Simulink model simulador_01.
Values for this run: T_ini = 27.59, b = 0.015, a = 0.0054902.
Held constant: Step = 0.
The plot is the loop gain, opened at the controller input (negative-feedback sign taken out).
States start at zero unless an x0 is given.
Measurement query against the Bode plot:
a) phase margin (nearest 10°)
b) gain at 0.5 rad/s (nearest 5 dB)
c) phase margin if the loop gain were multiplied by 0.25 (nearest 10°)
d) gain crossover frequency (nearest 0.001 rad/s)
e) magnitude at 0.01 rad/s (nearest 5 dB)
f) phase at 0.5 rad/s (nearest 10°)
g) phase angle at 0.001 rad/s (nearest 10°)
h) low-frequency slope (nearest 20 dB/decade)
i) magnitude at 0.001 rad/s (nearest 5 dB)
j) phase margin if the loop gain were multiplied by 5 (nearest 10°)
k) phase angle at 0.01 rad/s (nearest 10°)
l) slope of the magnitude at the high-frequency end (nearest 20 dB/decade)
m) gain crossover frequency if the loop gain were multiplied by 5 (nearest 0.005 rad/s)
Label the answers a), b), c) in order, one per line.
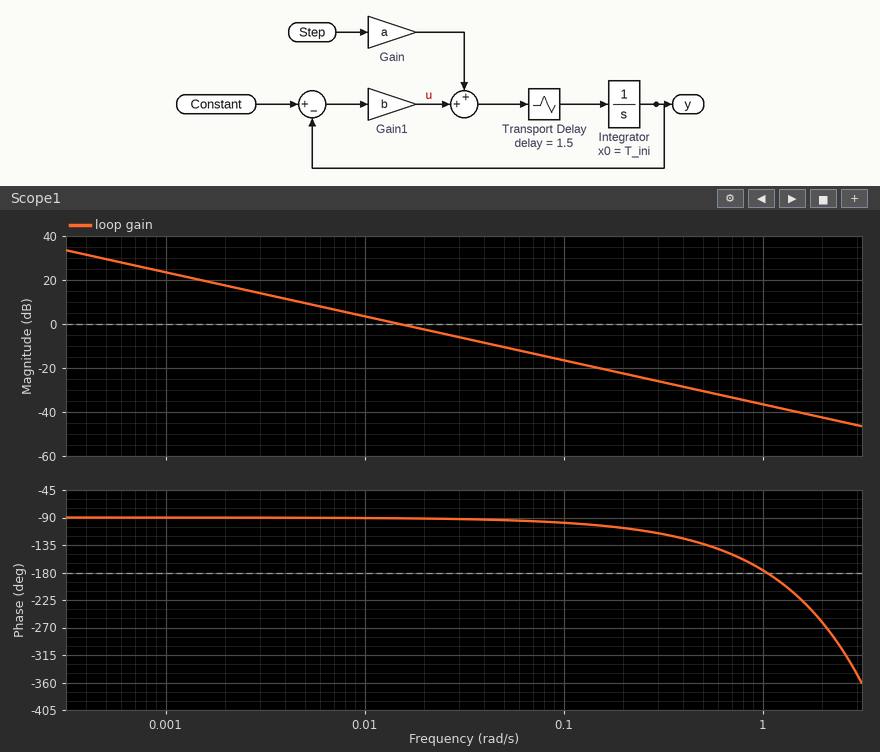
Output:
a) 90°
b) -30 dB
c) 90°
d) 0.015 rad/s
e) 5 dB
f) -130°
g) -90°
h) -20 dB/decade
i) 25 dB
j) 80°
k) -90°
l) -20 dB/decade
m) 0.075 rad/s
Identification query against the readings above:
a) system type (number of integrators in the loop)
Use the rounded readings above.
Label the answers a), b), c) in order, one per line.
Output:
a) 1
